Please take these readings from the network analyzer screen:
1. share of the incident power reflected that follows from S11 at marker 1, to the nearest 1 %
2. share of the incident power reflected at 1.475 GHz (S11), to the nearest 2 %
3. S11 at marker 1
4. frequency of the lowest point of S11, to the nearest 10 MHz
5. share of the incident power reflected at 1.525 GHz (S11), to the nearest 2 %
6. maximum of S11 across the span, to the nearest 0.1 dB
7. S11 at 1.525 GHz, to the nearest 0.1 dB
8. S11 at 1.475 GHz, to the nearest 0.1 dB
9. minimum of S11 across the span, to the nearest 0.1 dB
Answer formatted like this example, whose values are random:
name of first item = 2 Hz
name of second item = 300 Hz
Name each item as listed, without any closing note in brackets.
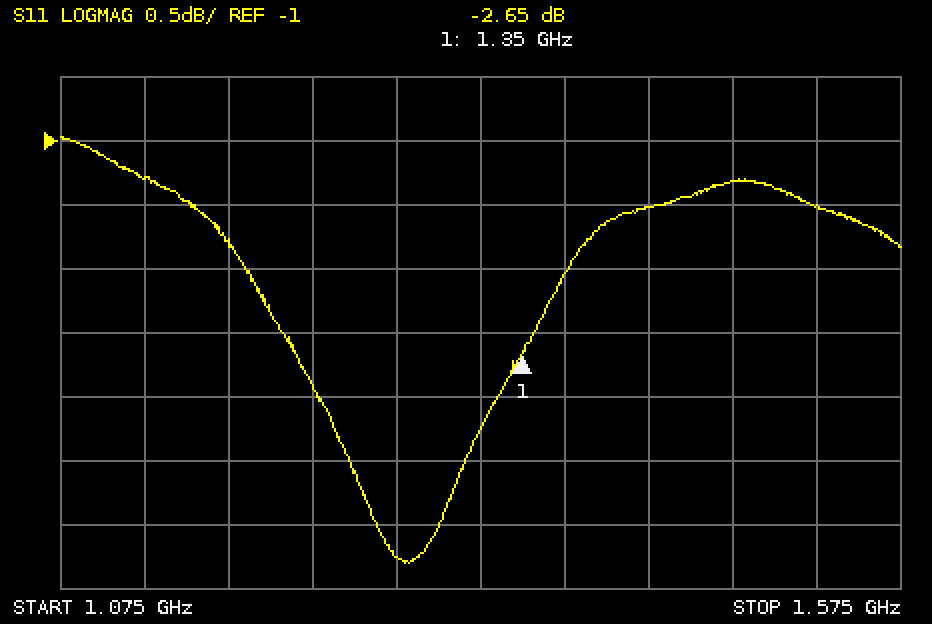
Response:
share of the incident power reflected that follows from S11 at marker 1, to the nearest 1 % = 54 %
share of the incident power reflected at 1.475 GHz (S11), to the nearest 2 % = 74 %
S11 at marker 1 = -2.65 dB
frequency of the lowest point of S11, to the nearest 10 MHz = 1.28 GHz
share of the incident power reflected at 1.525 GHz (S11), to the nearest 2 % = 70 %
maximum of S11 across the span, to the nearest 0.1 dB = -1.0 dB
S11 at 1.525 GHz, to the nearest 0.1 dB = -1.5 dB
S11 at 1.475 GHz, to the nearest 0.1 dB = -1.3 dB
minimum of S11 across the span, to the nearest 0.1 dB = -4.3 dB
